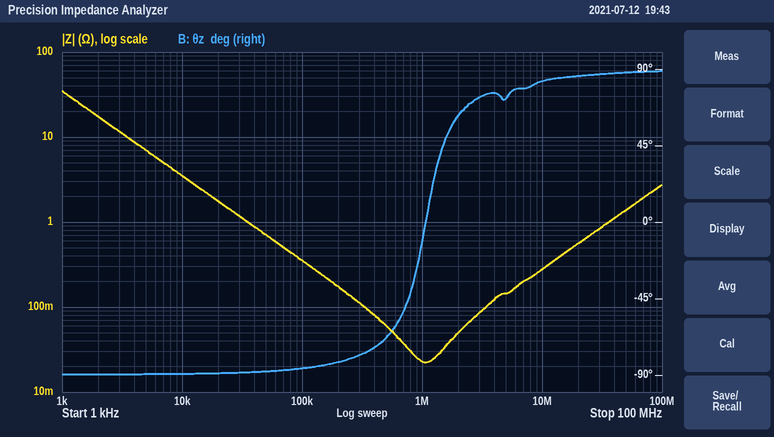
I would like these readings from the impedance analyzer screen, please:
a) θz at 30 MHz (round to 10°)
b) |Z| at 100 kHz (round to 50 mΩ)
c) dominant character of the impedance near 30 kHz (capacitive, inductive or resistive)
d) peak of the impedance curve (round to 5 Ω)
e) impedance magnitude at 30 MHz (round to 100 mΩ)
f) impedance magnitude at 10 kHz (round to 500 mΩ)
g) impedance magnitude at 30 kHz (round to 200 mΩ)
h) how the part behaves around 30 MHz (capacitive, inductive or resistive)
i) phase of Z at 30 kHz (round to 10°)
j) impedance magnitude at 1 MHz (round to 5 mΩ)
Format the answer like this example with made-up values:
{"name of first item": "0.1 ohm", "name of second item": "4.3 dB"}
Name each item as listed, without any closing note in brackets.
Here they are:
{"θz at 30 MHz": "90°", "|Z| at 100 kHz": "350 mΩ", "dominant character of the impedance near 30 kHz": "capacitive", "peak of the impedance curve": "35 Ω", "impedance magnitude at 30 MHz": "800 mΩ", "impedance magnitude at 10 kHz": "3.5 Ω", "impedance magnitude at 30 kHz": "1.2 Ω", "how the part behaves around 30 MHz": "inductive", "phase of Z at 30 kHz": "-90°", "impedance magnitude at 1 MHz": "25 mΩ"}
